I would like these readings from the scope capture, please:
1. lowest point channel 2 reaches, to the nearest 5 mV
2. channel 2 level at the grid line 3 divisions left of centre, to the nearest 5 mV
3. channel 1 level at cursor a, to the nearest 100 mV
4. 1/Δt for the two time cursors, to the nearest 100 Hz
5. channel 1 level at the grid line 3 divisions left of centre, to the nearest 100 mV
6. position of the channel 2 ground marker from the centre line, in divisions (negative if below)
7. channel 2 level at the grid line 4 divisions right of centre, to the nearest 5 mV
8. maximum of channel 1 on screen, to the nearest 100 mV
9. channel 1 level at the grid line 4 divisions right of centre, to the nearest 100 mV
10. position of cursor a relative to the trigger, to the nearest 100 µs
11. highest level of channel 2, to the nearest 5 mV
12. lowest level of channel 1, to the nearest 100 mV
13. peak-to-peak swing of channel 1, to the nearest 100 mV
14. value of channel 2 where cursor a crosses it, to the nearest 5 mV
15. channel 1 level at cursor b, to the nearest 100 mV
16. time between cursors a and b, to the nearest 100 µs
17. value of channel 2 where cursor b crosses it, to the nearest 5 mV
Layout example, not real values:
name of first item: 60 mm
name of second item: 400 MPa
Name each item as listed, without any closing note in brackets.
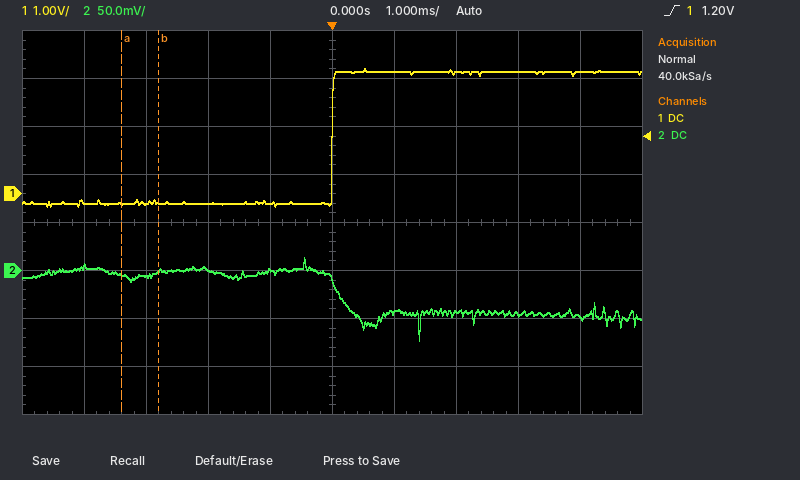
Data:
lowest point channel 2 reaches, to the nearest 5 mV: -75 mV
channel 2 level at the grid line 3 divisions left of centre, to the nearest 5 mV: -5 mV
channel 1 level at cursor a, to the nearest 100 mV: -200 mV
1/Δt for the two time cursors, to the nearest 100 Hz: 1.7 kHz
channel 1 level at the grid line 3 divisions left of centre, to the nearest 100 mV: -200 mV
position of the channel 2 ground marker from the centre line, in divisions: -1.0 div
channel 2 level at the grid line 4 divisions right of centre, to the nearest 5 mV: -50 mV
maximum of channel 1 on screen, to the nearest 100 mV: 2.6 V
channel 1 level at the grid line 4 divisions right of centre, to the nearest 100 mV: 2.5 V
position of cursor a relative to the trigger, to the nearest 100 µs: -3.4 ms
highest level of channel 2, to the nearest 5 mV: 15 mV
lowest level of channel 1, to the nearest 100 mV: -300 mV
peak-to-peak swing of channel 1, to the nearest 100 mV: 2.9 V
value of channel 2 where cursor a crosses it, to the nearest 5 mV: -5 mV
channel 1 level at cursor b, to the nearest 100 mV: -200 mV
time between cursors a and b, to the nearest 100 µs: 600 µs
value of channel 2 where cursor b crosses it, to the nearest 5 mV: 0 mV
